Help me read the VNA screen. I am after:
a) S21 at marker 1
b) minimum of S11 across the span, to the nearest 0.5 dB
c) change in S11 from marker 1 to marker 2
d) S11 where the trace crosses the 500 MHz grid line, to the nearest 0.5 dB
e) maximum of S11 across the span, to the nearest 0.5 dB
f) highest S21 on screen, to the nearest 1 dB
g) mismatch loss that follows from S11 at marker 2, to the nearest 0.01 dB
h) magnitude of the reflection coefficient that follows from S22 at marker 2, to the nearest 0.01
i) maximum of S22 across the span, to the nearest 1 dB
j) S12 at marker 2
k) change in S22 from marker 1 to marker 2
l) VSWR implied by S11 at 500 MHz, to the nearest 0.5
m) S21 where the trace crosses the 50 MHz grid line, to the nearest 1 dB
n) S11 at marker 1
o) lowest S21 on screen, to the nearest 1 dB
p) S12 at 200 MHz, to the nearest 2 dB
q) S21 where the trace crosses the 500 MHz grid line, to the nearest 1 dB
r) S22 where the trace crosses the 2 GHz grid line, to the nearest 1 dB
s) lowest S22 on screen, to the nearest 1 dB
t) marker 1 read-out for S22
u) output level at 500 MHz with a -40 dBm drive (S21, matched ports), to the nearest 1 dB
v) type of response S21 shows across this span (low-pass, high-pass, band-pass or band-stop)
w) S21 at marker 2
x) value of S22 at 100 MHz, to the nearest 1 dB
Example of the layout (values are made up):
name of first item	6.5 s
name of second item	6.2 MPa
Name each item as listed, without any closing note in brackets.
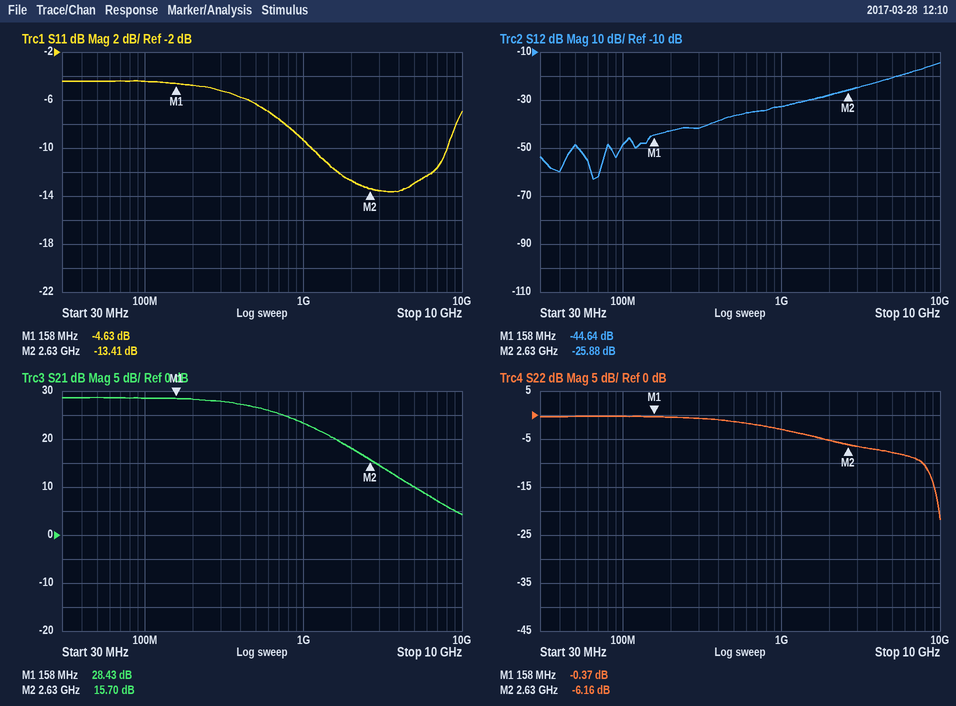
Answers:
S21 at marker 1	28.43 dB
minimum of S11 across the span, to the nearest 0.5 dB	-13.5 dB
change in S11 from marker 1 to marker 2	-8.78 dB
S11 where the trace crosses the 500 MHz grid line, to the nearest 0.5 dB	-6.5 dB
maximum of S11 across the span, to the nearest 0.5 dB	-4.5 dB
highest S21 on screen, to the nearest 1 dB	29 dB
mismatch loss that follows from S11 at marker 2, to the nearest 0.01 dB	0.20 dB
magnitude of the reflection coefficient that follows from S22 at marker 2, to the nearest 0.01	0.49
maximum of S22 across the span, to the nearest 1 dB	0 dB
S12 at marker 2	-25.88 dB
change in S22 from marker 1 to marker 2	-5.79 dB
VSWR implied by S11 at 500 MHz, to the nearest 0.5	3.0
S21 where the trace crosses the 50 MHz grid line, to the nearest 1 dB	29 dB
S11 at marker 1	-4.63 dB
lowest S21 on screen, to the nearest 1 dB	4 dB
S12 at 200 MHz, to the nearest 2 dB	-42 dB
S21 where the trace crosses the 500 MHz grid line, to the nearest 1 dB	27 dB
S22 where the trace crosses the 2 GHz grid line, to the nearest 1 dB	-5 dB
lowest S22 on screen, to the nearest 1 dB	-22 dB
marker 1 read-out for S22	-0.37 dB
output level at 500 MHz with a -40 dBm drive (S21, matched ports), to the nearest 1 dB	-13 dBm
type of response S21 shows across this span	low-pass
S21 at marker 2	15.70 dB
value of S22 at 100 MHz, to the nearest 1 dB	0 dB
